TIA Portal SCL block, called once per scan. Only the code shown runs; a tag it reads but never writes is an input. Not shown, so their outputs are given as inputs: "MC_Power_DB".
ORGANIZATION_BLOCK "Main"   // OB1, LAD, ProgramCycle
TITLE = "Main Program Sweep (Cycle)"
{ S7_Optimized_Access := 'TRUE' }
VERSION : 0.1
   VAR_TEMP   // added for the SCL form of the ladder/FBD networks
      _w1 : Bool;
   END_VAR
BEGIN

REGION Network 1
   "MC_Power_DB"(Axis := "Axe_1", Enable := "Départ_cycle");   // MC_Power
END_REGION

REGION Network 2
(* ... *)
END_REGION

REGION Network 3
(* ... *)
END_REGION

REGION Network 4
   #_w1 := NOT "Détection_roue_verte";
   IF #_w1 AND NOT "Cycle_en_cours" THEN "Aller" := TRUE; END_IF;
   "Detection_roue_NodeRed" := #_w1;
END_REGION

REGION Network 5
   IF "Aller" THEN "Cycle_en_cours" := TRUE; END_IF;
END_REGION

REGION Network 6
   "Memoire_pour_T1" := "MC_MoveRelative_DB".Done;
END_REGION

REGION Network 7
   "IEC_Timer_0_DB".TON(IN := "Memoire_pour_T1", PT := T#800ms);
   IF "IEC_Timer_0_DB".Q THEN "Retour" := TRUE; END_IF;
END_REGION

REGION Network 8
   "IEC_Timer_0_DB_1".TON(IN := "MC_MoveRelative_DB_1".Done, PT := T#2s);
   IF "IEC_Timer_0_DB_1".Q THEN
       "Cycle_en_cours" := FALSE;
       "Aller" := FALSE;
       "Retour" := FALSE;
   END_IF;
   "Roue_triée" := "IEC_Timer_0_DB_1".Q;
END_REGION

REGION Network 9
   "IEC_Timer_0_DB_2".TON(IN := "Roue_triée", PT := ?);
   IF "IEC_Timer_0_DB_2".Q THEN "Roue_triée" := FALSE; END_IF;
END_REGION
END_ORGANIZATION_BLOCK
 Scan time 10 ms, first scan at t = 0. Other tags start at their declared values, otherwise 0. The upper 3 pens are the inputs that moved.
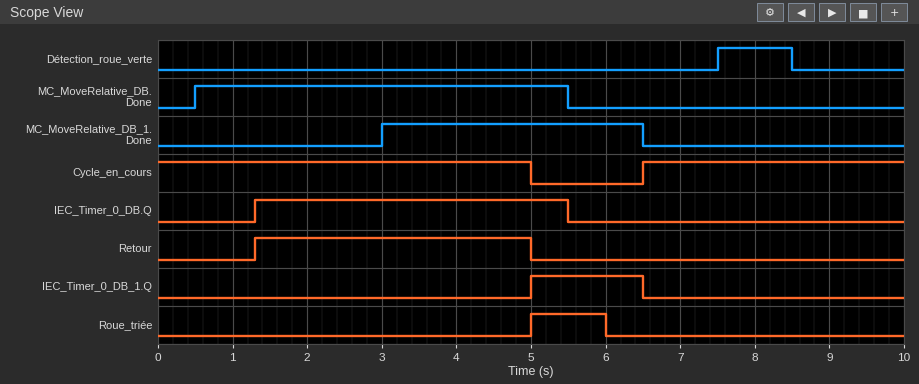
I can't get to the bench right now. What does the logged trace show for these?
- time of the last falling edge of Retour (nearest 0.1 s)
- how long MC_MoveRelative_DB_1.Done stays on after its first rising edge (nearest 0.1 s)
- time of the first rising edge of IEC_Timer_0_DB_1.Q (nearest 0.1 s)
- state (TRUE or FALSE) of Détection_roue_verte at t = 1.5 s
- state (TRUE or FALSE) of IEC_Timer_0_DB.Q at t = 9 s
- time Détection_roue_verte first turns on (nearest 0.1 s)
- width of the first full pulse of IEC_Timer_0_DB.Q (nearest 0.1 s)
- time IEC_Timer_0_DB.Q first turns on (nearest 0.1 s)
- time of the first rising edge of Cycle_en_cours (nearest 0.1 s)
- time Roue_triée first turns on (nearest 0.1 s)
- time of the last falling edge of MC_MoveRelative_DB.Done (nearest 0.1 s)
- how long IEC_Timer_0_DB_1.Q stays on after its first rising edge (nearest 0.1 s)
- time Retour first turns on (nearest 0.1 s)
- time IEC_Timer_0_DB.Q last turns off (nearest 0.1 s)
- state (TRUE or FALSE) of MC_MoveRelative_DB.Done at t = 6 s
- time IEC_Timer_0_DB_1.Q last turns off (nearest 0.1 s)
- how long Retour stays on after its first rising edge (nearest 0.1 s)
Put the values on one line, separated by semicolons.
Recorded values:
5.0 s; 3.5 s; 5.0 s; FALSE; FALSE; 7.5 s; 4.2 s; 1.3 s; 6.5 s; 5.0 s; 5.5 s; 1.5 s; 1.3 s; 5.5 s; FALSE; 6.5 s; 3.7 s
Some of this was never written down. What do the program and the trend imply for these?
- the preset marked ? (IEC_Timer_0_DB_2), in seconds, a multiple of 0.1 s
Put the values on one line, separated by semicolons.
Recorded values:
1.0 s
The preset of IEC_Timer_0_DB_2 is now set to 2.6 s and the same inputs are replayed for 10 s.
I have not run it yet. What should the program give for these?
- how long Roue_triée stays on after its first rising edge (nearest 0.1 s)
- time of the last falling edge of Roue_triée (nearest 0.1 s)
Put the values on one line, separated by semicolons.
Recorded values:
1.5 s; 6.5 s
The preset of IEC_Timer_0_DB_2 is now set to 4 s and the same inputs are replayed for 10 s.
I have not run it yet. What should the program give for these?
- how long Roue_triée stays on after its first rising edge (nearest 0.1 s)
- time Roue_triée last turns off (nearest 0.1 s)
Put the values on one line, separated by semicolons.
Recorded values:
1.5 s; 6.5 s
